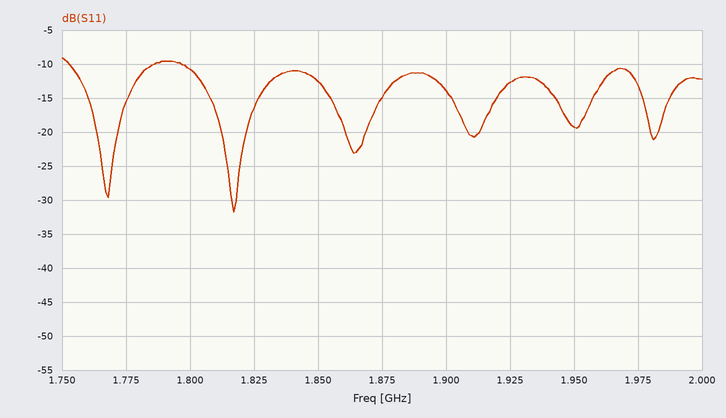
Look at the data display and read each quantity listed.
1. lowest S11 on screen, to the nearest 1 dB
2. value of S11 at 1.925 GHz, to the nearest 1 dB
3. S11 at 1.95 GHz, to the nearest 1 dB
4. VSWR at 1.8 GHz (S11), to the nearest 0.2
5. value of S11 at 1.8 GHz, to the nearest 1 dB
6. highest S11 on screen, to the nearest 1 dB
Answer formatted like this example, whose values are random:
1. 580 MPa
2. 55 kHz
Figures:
1. -32 dB
2. -13 dB
3. -19 dB
4. 1.8
5. -11 dB
6. -9 dB
